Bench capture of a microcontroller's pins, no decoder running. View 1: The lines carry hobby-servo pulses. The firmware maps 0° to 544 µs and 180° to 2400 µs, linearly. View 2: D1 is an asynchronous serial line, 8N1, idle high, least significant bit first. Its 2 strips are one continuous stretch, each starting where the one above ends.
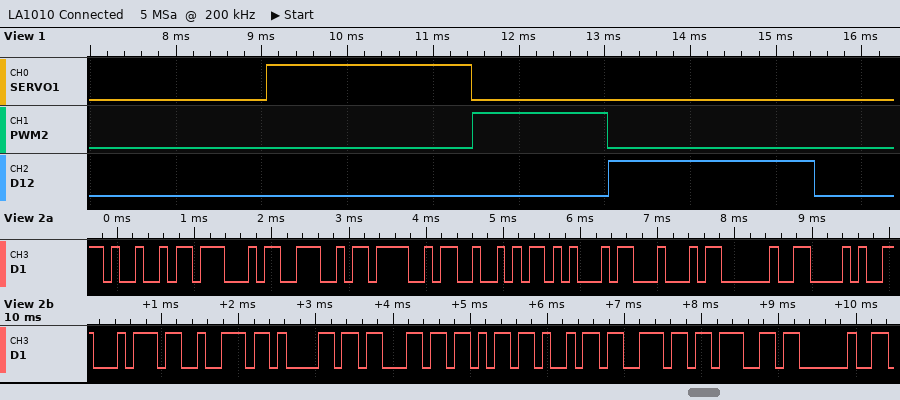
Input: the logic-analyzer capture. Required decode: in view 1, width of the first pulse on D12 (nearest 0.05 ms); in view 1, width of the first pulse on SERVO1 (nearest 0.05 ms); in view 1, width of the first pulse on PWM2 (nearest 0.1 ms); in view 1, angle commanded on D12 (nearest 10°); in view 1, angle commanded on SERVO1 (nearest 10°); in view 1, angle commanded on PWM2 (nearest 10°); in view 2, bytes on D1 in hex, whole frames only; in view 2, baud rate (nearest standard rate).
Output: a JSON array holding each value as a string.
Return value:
["2.40 ms", "2.40 ms", "1.6 ms", "180°", "180°", "100°", "49 47 4E 4F 52 45 44 20 28 74 72 61 63 6B 69 6E 67 20", "9600 baud"]
